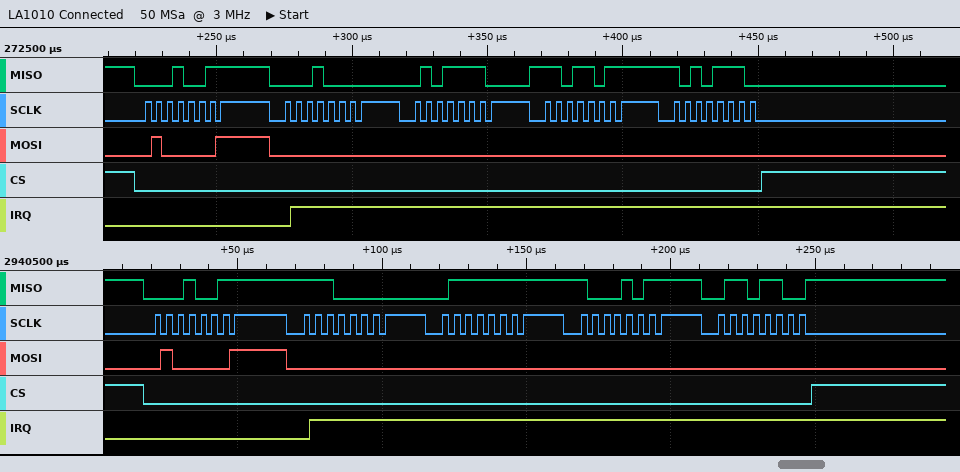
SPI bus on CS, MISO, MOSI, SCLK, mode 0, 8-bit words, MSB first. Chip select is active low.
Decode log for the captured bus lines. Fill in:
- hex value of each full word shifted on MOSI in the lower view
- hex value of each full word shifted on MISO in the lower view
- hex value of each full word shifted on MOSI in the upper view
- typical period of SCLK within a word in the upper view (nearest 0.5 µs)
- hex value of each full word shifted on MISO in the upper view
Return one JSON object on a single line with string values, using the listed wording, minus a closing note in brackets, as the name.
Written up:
{"hex value of each full word shifted on MOSI in the lower view": "41, 00, 00, 00, 00", "hex value of each full word shifted on MISO in the lower view": "13, E0, 7F, 8B, 6C", "hex value of each full word shifted on MOSI in the upper view": "41, 00, 00, 00, 00", "typical period of SCLK within a word in the upper view": "4 µs", "hex value of each full word shifted on MISO in the upper view": "13, 10, 5E, DB, AE"}
